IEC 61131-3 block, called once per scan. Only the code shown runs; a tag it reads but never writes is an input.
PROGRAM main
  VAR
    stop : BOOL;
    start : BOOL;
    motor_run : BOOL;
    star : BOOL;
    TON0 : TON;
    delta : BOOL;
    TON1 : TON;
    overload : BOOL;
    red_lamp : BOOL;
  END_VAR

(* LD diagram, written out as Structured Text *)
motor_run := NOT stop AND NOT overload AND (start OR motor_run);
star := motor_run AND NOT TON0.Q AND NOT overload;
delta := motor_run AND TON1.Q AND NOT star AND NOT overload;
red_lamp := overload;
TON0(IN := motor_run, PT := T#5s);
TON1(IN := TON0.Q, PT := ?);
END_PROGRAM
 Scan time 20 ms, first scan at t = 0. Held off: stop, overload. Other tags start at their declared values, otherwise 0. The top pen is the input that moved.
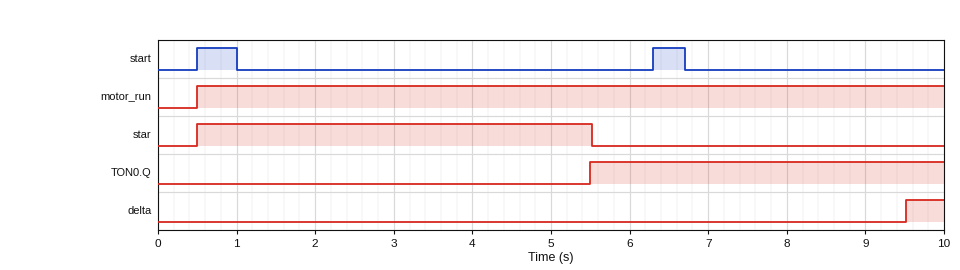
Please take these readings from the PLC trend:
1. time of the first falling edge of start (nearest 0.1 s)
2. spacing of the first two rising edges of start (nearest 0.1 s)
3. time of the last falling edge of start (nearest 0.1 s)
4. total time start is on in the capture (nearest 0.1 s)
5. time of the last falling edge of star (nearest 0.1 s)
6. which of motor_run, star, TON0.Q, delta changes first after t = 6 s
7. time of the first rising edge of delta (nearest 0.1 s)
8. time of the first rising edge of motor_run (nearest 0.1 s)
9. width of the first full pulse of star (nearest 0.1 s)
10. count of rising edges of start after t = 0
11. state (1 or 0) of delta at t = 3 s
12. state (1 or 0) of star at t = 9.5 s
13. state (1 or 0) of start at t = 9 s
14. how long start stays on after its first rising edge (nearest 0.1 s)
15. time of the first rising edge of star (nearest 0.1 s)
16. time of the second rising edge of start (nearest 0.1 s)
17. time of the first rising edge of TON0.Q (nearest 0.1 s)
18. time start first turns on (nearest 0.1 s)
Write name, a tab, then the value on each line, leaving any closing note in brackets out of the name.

time of the first falling edge of start	1.0 s
spacing of the first two rising edges of start	5.8 s
time of the last falling edge of start	6.7 s
total time start is on in the capture	0.9 s
time of the last falling edge of star	5.5 s
which of motor_run, star, TON0.Q, delta changes first after t = 6 s	delta
time of the first rising edge of delta	9.5 s
time of the first rising edge of motor_run	0.5 s
width of the first full pulse of star	5.0 s
count of rising edges of start after t = 0	2
state (1 or 0) of delta at t = 3 s	0
state (1 or 0) of star at t = 9.5 s	0
state (1 or 0) of start at t = 9 s	0
how long start stays on after its first rising edge	0.5 s
time of the first rising edge of star	0.5 s
time of the second rising edge of start	6.3 s
time of the first rising edge of TON0.Q	5.5 s
time start first turns on	0.5 s
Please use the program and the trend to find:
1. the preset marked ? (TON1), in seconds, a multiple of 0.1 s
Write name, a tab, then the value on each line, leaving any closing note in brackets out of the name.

the preset marked ? (TON1), in seconds, a multiple of 0.1 s	4.0 s
